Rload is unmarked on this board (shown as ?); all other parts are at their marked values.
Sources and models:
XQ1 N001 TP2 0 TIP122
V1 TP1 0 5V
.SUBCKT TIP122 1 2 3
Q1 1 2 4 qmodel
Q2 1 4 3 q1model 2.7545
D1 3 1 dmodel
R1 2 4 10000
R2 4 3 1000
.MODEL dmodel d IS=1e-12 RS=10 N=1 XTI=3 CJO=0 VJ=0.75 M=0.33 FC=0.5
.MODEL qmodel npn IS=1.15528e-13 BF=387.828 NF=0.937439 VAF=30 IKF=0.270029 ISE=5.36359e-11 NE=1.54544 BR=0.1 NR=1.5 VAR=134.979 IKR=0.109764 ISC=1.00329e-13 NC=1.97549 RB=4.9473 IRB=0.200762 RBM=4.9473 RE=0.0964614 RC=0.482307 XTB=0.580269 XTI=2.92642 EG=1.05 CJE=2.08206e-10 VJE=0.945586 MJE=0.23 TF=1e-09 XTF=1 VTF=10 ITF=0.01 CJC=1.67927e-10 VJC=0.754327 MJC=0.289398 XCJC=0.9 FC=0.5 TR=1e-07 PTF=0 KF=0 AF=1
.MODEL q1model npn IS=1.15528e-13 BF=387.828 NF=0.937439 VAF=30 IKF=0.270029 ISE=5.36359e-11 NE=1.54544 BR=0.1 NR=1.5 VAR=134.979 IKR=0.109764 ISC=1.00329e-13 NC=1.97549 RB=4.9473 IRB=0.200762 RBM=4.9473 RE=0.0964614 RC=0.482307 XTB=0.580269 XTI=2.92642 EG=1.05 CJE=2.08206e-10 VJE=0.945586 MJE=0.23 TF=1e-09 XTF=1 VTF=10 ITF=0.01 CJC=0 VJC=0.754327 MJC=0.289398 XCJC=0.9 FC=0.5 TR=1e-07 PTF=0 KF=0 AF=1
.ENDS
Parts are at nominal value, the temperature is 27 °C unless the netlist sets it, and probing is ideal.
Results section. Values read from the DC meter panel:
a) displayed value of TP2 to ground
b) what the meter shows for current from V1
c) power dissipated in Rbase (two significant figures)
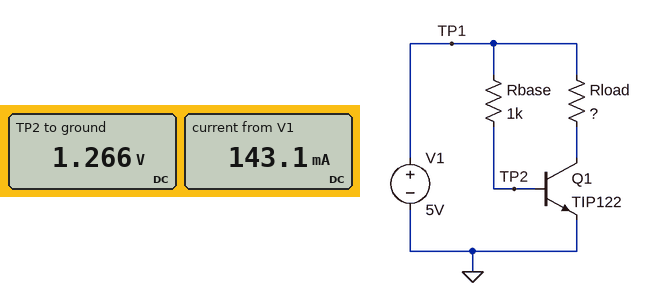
1.266 V
143.1 mA
14 mW
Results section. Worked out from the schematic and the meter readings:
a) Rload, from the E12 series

33 Ω
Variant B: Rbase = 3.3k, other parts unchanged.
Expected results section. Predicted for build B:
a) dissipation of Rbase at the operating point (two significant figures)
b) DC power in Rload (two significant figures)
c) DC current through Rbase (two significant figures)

4.3 mW
630 mW
1.1 mA
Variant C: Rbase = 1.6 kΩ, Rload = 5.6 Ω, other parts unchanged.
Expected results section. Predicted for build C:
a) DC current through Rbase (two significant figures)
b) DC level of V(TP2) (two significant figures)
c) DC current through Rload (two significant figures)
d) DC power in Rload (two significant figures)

2.3 mA
1.4 V
790 mA
3.5 W
